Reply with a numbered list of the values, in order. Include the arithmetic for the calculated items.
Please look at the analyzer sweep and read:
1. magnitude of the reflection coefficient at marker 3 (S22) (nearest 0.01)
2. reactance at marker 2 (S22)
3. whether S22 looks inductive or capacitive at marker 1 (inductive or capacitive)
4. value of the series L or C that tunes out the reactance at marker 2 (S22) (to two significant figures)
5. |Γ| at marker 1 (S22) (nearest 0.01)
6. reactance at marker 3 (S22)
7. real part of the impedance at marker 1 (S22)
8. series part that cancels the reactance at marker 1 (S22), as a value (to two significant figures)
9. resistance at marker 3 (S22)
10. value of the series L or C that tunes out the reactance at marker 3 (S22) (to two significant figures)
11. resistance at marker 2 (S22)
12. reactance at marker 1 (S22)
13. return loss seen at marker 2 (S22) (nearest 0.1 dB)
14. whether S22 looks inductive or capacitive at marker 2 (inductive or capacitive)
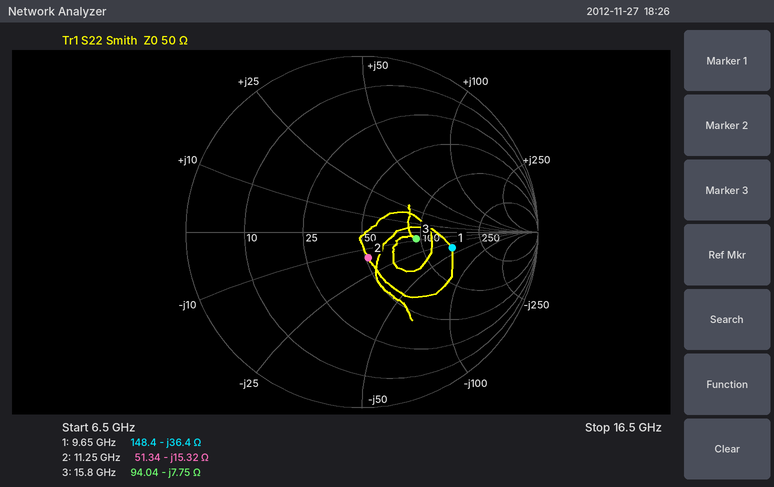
1. 0.31
2. -15.32 Ω
3. capacitive
4. L = 15.32 Ω/(2π × 11.25 GHz) ≈ 217 pH, so 220 pH to two significant figures
5. 0.52
6. -7.75 Ω
7. 148.4 Ω
8. L = 36.4 Ω/(2π × 9.65 GHz) ≈ 600 pH
9. 94.04 Ω
10. L = 7.75 Ω/(2π × 15.8 GHz) ≈ 78 pH
11. 51.34 Ω
12. -36.4 Ω
13. 16.5 dB
14. capacitive
